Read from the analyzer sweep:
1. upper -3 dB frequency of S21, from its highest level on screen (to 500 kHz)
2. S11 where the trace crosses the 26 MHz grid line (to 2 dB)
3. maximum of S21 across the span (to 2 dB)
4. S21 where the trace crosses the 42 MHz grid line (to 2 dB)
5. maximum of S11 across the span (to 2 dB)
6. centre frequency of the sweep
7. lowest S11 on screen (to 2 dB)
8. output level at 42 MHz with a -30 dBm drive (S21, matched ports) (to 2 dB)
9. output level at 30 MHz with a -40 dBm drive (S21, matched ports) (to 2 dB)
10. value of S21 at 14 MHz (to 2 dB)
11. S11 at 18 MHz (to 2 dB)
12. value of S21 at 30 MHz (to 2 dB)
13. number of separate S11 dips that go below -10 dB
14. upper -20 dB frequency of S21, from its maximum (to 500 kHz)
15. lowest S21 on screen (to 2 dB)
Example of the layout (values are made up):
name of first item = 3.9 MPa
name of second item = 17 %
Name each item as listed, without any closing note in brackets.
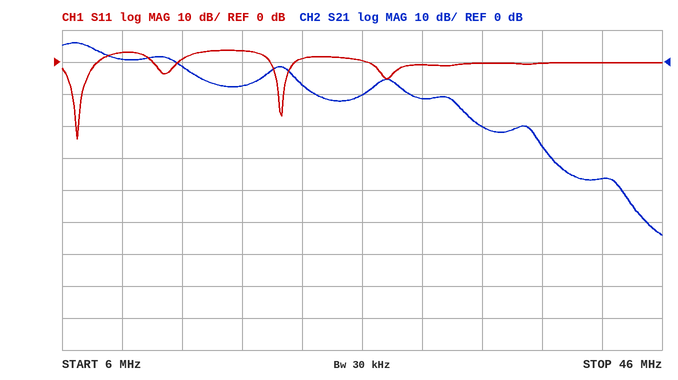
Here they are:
upper -3 dB frequency of S21, from its highest level on screen = 8.5 MHz
S11 where the trace crosses the 26 MHz grid line = 0 dB
maximum of S21 across the span = 6 dB
S21 where the trace crosses the 42 MHz grid line = -36 dB
maximum of S11 across the span = 4 dB
centre frequency of the sweep = 26 MHz
lowest S11 on screen = -24 dB
output level at 42 MHz with a -30 dBm drive (S21, matched ports) = -66 dBm
output level at 30 MHz with a -40 dBm drive (S21, matched ports) = -52 dBm
value of S21 at 14 MHz = -2 dB
S11 at 18 MHz = 4 dB
value of S21 at 30 MHz = -12 dB
number of separate S11 dips that go below -10 dB = 2
upper -20 dB frequency of S21, from its maximum = 32.5 MHz
lowest S21 on screen = -54 dB
